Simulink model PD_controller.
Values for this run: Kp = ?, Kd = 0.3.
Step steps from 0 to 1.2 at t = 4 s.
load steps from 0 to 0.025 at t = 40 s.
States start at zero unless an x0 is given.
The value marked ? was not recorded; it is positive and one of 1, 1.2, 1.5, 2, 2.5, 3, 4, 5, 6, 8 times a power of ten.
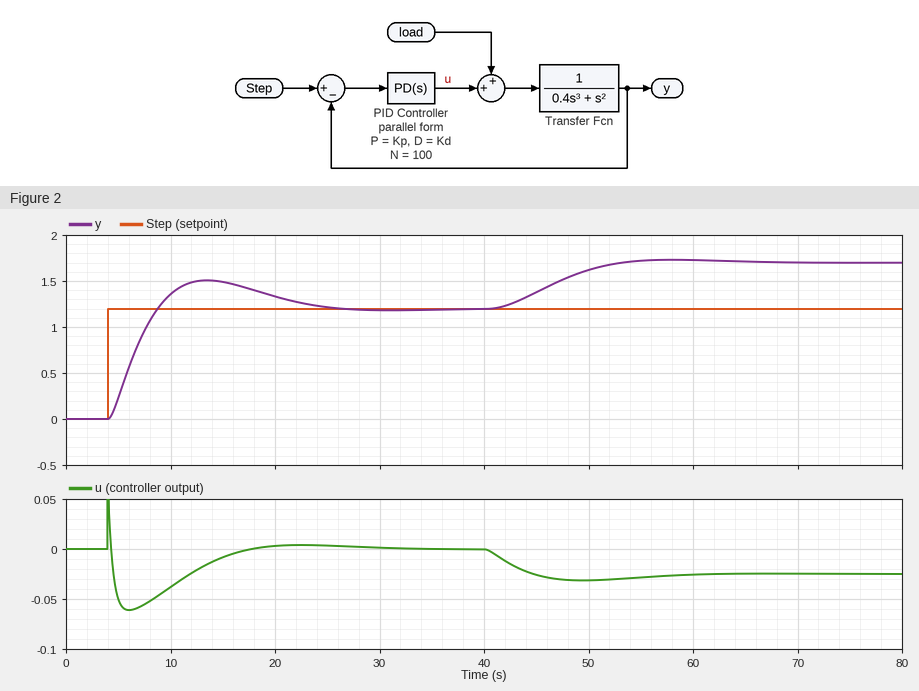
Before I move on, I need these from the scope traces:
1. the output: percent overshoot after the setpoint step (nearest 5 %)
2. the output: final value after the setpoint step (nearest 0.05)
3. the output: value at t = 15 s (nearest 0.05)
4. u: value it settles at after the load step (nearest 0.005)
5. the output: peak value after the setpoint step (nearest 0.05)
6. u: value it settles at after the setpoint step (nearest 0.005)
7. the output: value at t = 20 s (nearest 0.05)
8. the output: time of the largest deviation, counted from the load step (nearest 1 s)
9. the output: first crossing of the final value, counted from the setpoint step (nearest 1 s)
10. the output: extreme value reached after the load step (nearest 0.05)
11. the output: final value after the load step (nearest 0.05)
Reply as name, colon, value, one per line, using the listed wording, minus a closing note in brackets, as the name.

the output: percent overshoot after the setpoint step: 25 %
the output: final value after the setpoint step: 1.20
the output: value at t = 15 s: 1.50
u: value it settles at after the load step: -0.025
the output: peak value after the setpoint step: 1.50
u: value it settles at after the setpoint step: 0.000
the output: value at t = 20 s: 1.35
the output: time of the largest deviation, counted from the load step: 18 s
the output: first crossing of the final value, counted from the setpoint step: 5 s
the output: extreme value reached after the load step: 1.75
the output: final value after the load step: 1.70
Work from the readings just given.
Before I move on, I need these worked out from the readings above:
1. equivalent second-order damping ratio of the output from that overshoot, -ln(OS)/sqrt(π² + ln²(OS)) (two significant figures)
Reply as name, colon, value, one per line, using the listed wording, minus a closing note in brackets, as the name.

equivalent second-order damping ratio of the output from that overshoot, -ln(OS)/sqrt(π² + ln²(OS)): 0.40
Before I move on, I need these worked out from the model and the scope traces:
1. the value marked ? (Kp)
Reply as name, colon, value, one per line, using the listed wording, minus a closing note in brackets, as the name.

the value marked ?: 0.05
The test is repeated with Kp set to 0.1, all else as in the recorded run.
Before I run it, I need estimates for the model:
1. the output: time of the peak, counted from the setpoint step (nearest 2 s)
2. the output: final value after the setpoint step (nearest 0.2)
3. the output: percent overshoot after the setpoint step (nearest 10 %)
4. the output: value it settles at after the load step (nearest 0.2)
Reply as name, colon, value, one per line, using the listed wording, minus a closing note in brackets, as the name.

the output: time of the peak, counted from the setpoint step: 8 s
the output: final value after the setpoint step: 1.2
the output: percent overshoot after the setpoint step: 40 %
the output: value it settles at after the load step: 1.4
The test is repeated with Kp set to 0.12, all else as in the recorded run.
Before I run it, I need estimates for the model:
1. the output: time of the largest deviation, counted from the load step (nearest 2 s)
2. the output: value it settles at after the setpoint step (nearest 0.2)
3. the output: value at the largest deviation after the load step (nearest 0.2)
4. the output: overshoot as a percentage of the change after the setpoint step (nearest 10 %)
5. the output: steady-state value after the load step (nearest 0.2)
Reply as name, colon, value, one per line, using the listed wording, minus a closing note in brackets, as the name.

the output: time of the largest deviation, counted from the load step: 10 s
the output: value it settles at after the setpoint step: 1.2
the output: value at the largest deviation after the load step: 1.4
the output: overshoot as a percentage of the change after the setpoint step: 40 %
the output: steady-state value after the load step: 1.4
